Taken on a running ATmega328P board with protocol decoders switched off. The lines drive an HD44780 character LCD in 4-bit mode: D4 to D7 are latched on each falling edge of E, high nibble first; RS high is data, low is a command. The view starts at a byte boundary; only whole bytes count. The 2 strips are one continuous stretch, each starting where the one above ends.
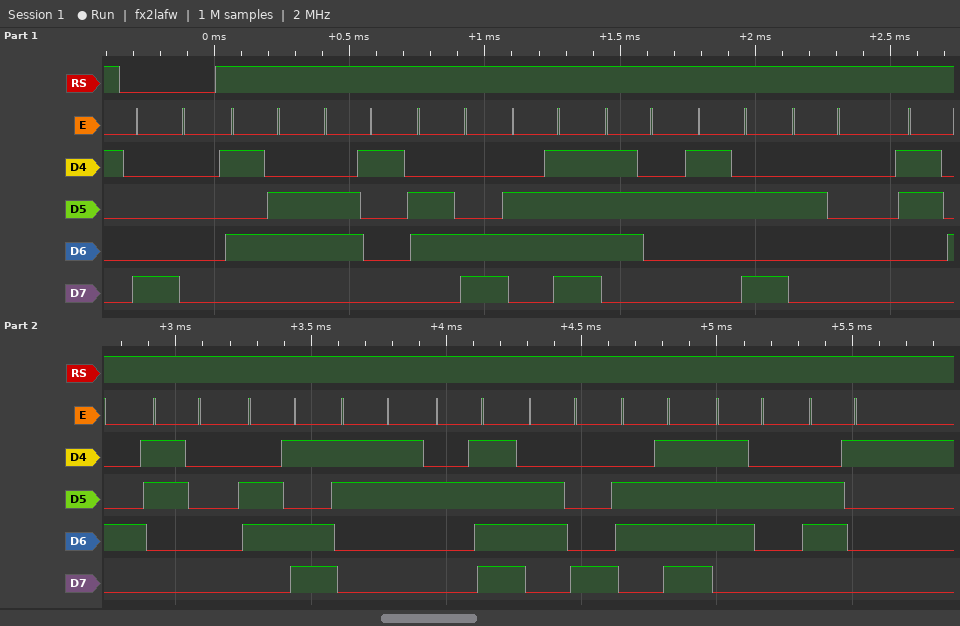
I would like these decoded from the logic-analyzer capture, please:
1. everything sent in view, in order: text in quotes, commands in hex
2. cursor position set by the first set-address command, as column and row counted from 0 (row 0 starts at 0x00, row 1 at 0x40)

0x80 "Valor: 40m3/hora"
column 0, row 0
